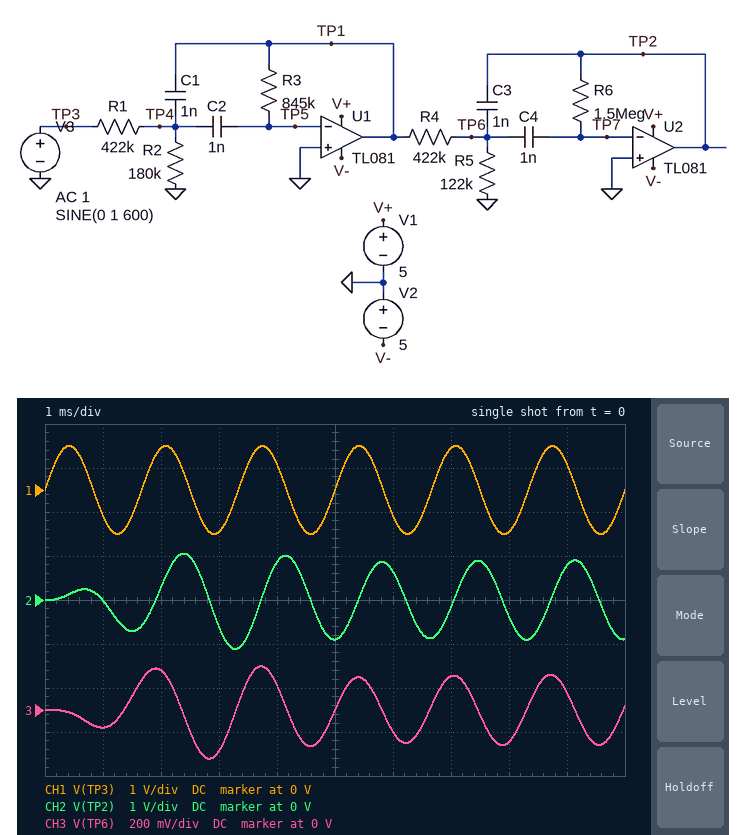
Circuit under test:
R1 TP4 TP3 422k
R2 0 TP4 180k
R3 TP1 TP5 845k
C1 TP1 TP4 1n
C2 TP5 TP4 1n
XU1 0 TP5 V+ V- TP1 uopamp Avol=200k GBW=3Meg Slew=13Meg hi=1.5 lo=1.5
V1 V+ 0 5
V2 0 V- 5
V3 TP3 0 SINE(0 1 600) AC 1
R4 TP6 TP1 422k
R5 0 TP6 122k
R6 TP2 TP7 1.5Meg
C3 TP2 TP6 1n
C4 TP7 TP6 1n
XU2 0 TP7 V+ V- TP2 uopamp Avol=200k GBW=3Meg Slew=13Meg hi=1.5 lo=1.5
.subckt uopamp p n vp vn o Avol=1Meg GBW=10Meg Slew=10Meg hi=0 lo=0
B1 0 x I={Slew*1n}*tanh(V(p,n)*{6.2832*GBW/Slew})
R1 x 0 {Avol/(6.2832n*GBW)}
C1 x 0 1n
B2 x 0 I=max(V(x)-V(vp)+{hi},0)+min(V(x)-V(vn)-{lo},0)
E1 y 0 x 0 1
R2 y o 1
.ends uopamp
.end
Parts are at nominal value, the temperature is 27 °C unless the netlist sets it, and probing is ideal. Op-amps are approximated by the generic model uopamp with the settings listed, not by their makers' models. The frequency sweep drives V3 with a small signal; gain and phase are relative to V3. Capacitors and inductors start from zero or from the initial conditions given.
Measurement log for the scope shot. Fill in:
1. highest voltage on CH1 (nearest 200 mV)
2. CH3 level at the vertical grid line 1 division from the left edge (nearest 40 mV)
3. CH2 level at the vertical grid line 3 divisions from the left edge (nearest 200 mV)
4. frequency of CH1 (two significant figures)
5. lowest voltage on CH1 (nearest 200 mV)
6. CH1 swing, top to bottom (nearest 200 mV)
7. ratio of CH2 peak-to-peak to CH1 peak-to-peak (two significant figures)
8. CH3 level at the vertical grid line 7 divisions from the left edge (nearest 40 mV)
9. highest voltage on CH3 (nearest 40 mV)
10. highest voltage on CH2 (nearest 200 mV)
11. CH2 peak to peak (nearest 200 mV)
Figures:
1.0 V
-80 mV
-600 mV
600 Hz
-1.0 V
2.0 V
1.1
160 mV
200 mV
1.0 V
2.2 V
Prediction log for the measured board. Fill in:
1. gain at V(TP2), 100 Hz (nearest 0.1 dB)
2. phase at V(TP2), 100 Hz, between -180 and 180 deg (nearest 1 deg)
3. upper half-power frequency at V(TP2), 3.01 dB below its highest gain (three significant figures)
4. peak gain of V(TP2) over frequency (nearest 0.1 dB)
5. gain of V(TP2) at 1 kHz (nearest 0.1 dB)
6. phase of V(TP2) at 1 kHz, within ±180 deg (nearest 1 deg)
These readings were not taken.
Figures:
-28.8 dB
163 deg
544 Hz
4.6 dB
-14.1 dB
-139 deg
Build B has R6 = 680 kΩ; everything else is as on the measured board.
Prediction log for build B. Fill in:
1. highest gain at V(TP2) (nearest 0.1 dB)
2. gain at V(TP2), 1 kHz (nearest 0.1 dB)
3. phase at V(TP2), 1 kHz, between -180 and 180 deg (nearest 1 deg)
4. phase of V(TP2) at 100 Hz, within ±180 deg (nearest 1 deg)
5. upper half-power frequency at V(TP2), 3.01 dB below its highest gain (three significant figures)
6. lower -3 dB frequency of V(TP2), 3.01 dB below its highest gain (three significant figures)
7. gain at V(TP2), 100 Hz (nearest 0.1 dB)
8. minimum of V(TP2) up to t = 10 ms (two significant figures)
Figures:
-2.8 dB
-13.2 dB
-116 deg
164 deg
727 Hz
423 Hz
-35.9 dB
-710 mV
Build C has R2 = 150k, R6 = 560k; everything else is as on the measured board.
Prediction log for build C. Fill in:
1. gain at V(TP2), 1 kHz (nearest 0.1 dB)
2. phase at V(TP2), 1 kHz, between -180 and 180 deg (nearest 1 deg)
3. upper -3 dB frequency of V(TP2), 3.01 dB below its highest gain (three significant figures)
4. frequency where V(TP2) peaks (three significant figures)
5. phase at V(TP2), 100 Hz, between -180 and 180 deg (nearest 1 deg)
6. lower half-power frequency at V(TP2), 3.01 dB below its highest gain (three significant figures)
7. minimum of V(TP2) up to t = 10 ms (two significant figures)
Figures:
-13.0 dB
-105 deg
784 Hz
588 Hz
165 deg
447 Hz
-590 mV
